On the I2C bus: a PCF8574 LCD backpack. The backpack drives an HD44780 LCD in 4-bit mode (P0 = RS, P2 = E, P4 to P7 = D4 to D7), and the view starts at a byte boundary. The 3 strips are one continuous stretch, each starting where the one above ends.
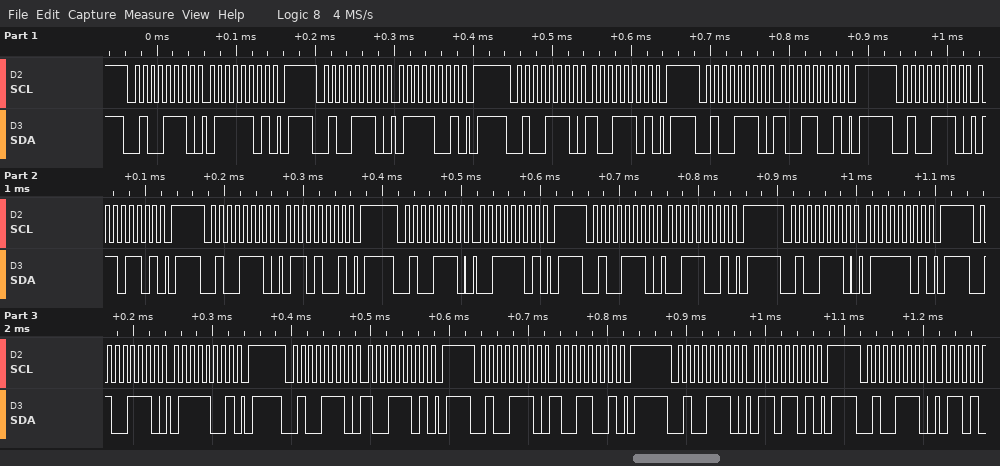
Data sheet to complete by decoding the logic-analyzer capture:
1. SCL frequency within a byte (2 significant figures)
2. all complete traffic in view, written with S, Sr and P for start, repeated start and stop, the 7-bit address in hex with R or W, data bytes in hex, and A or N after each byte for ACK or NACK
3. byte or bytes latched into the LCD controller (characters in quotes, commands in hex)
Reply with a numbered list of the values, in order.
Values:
1. 100 kHz
2. S 27W A 7D A P S 27W A 79 A P S 27W A 9D A P S 27W A 99 A P S 27W A 6D A P S 27W A 69 A P S 27W A 3D A P S 27W A 39 A P S 27W A 7D A P S 27W A 79 A P S 27W A 9D A P S 27W A 99 A P S 27W A 6D A P S 27W A
3. 'y' 'c' 'y'
